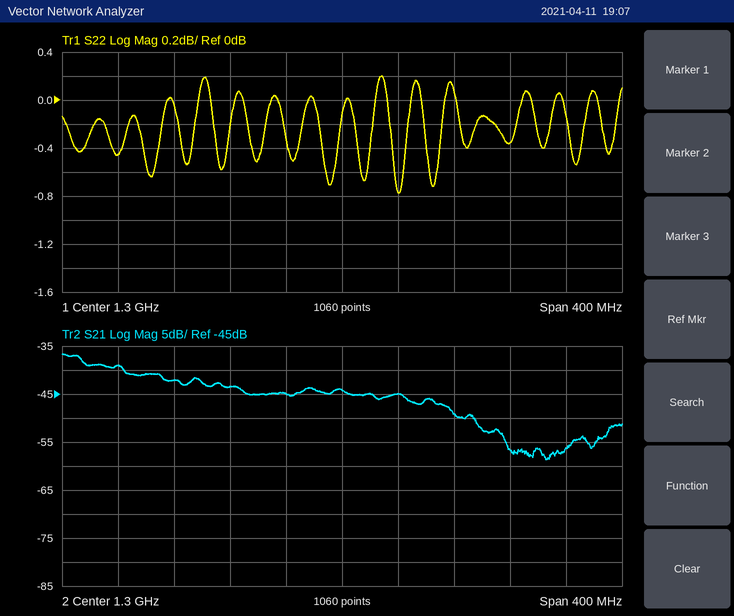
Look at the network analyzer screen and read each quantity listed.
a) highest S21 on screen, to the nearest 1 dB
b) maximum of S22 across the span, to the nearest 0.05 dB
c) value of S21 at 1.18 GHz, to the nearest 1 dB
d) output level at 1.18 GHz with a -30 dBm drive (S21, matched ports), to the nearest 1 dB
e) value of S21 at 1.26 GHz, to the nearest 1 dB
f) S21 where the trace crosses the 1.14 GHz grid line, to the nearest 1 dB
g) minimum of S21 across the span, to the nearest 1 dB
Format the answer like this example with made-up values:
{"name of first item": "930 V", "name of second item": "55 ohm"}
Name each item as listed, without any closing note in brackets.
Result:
{"highest S21 on screen, to the nearest 1 dB": "-37 dB", "maximum of S22 across the span, to the nearest 0.05 dB": "0.20 dB", "value of S21 at 1.18 GHz, to the nearest 1 dB": "-42 dB", "output level at 1.18 GHz with a -30 dBm drive (S21, matched ports), to the nearest 1 dB": "-72 dBm", "value of S21 at 1.26 GHz, to the nearest 1 dB": "-45 dB", "S21 where the trace crosses the 1.14 GHz grid line, to the nearest 1 dB": "-39 dB", "minimum of S21 across the span, to the nearest 1 dB": "-59 dB"}
